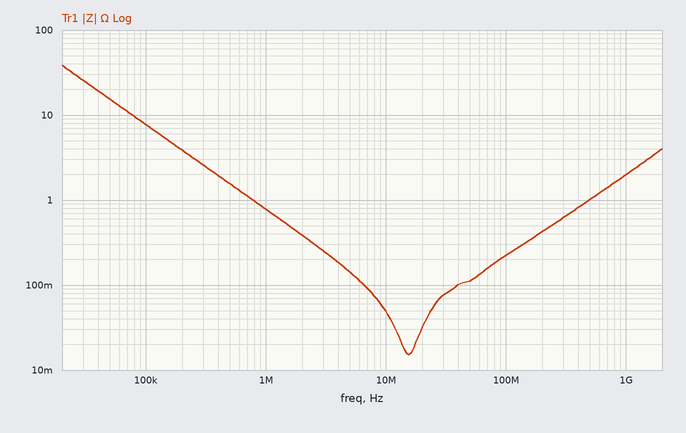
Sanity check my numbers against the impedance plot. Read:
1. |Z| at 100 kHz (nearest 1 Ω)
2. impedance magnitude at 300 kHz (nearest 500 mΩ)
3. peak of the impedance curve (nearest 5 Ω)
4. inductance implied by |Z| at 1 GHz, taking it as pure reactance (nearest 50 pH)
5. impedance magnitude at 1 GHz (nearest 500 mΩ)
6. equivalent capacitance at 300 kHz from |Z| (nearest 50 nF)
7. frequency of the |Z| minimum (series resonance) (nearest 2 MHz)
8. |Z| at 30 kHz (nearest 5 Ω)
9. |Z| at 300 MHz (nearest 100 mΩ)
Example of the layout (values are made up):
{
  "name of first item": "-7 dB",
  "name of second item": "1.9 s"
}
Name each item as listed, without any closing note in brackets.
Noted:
{
  "|Z| at 100 kHz": "8 Ω",
  "impedance magnitude at 300 kHz": "2.5 Ω",
  "peak of the impedance curve": "40 Ω",
  "inductance implied by |Z| at 1 GHz, taking it as pure reactance": "300 pH",
  "impedance magnitude at 1 GHz": "2.0 Ω",
  "equivalent capacitance at 300 kHz from |Z|": "200 nF",
  "frequency of the |Z| minimum (series resonance)": "16 MHz",
  "|Z| at 30 kHz": "25 Ω",
  "|Z| at 300 MHz": "600 mΩ"
}
